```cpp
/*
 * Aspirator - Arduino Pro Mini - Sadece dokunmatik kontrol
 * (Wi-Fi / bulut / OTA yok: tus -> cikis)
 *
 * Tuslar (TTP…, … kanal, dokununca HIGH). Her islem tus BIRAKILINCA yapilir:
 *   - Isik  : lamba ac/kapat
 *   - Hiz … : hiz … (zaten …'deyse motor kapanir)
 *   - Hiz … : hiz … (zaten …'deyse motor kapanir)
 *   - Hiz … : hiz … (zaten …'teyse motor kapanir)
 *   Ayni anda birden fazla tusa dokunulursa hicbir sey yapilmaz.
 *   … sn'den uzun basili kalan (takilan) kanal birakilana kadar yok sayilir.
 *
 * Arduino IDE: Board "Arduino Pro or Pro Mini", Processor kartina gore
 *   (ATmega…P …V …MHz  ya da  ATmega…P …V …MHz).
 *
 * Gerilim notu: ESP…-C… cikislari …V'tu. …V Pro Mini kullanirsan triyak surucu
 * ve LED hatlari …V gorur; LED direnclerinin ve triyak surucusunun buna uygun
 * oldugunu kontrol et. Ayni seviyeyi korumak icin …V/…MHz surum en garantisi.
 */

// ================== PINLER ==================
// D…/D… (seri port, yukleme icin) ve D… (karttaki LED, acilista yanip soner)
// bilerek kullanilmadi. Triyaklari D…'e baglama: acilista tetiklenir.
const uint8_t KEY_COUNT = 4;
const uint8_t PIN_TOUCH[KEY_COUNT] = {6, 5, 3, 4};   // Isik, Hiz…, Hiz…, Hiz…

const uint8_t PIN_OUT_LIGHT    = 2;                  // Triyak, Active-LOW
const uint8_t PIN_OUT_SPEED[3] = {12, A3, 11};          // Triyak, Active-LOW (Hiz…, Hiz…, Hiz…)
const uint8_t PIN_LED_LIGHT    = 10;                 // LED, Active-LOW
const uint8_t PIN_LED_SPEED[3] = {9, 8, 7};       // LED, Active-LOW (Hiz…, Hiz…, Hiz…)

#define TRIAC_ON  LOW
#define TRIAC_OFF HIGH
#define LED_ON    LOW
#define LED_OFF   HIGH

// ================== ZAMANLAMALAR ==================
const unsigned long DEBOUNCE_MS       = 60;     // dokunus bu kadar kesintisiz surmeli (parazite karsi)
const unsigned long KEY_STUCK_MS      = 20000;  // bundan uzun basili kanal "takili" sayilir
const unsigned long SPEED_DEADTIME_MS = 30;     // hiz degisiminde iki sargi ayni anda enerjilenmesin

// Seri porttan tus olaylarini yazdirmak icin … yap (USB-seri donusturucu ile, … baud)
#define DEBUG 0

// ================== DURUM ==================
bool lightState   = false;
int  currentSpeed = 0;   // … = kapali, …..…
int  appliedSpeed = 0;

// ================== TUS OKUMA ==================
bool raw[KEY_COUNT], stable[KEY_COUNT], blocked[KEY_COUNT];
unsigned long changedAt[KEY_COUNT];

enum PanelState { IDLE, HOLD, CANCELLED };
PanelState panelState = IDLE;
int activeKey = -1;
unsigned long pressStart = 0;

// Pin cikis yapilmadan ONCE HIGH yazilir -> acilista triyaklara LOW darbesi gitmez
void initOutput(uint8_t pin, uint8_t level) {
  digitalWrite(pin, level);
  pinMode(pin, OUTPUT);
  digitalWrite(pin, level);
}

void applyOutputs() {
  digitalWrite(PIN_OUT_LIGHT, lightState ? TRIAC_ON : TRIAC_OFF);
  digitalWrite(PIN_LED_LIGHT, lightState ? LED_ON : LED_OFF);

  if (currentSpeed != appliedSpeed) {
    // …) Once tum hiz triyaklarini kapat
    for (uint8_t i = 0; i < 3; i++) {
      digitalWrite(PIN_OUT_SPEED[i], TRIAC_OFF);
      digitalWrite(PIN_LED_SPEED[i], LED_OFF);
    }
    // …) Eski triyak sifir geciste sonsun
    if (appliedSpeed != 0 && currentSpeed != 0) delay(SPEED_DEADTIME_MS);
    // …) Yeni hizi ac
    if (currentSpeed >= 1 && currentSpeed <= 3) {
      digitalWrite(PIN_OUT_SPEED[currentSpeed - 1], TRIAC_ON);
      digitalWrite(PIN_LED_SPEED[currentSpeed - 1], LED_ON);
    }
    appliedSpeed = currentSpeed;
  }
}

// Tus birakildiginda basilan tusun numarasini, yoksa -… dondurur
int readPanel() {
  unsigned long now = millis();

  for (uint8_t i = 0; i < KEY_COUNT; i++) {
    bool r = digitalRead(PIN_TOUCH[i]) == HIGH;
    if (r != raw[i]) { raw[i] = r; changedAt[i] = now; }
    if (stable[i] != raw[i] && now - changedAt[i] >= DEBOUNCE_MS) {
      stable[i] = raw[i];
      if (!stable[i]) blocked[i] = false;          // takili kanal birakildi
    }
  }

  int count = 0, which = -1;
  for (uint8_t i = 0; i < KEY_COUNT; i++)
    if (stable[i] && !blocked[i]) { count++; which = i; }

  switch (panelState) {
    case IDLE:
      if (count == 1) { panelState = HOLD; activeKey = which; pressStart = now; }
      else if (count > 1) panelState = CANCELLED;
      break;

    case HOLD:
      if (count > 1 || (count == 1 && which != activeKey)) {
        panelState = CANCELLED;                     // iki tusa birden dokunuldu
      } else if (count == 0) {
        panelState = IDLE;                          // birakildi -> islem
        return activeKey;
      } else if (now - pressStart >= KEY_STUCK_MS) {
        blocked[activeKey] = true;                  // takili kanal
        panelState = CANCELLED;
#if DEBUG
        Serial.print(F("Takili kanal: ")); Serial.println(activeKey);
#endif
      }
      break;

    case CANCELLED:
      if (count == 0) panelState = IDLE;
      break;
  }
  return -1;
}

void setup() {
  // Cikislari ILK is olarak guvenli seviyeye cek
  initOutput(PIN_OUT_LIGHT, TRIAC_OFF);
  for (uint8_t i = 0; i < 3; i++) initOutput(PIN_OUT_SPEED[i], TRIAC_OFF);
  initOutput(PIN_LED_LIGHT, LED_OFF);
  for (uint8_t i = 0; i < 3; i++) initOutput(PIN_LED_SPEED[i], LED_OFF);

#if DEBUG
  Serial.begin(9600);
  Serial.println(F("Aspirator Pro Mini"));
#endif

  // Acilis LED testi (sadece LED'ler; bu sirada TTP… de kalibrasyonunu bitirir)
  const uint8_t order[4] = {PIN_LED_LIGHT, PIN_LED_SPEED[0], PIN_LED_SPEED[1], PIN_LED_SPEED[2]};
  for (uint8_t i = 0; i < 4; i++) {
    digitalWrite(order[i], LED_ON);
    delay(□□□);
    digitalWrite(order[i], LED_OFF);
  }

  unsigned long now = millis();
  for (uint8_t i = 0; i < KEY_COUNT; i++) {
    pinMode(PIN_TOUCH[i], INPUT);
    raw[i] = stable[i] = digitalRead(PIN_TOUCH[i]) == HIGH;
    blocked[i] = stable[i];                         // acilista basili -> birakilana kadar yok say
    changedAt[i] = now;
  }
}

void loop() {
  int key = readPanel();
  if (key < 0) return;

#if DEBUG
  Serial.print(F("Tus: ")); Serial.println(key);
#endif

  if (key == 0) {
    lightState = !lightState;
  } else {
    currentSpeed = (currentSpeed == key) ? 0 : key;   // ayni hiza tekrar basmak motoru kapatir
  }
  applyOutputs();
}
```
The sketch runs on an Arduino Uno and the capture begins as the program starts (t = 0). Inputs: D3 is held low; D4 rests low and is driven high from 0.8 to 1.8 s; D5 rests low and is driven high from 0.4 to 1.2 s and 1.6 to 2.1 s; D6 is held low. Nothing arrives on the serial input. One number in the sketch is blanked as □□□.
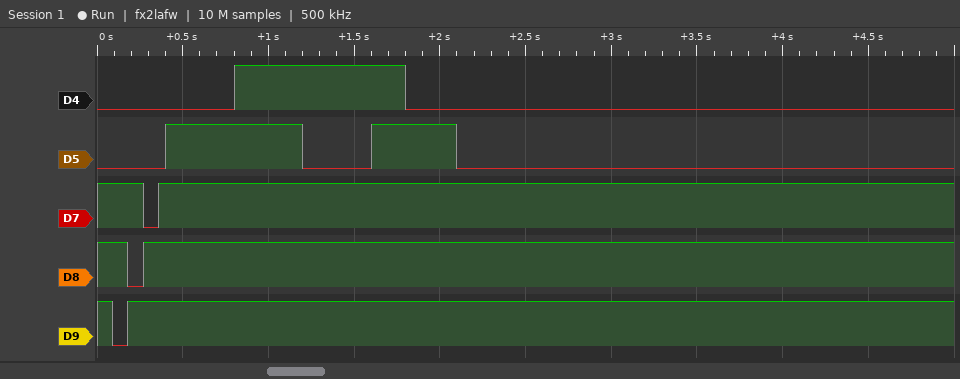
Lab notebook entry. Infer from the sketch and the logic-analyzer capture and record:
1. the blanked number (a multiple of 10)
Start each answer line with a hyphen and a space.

- 90
